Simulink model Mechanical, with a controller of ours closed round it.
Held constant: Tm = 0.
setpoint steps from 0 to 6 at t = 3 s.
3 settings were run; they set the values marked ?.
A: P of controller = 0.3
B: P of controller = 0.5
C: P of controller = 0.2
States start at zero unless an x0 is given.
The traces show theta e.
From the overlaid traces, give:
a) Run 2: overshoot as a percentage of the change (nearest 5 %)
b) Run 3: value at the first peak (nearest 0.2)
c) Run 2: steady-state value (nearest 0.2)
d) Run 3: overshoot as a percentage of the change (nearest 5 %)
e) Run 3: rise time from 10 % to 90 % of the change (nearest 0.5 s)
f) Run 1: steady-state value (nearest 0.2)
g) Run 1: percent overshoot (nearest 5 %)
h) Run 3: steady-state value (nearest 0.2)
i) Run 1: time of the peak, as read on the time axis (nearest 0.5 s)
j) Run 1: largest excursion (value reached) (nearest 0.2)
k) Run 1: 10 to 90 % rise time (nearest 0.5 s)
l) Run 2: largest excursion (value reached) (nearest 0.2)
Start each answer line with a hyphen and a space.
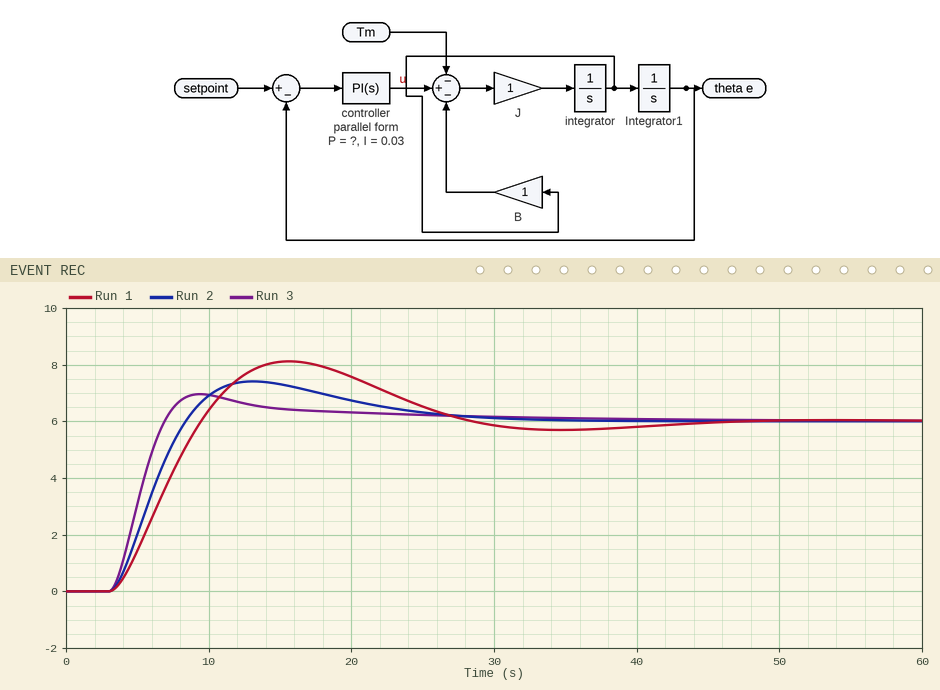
- 25 %
- 7.0
- 6.0
- 15 %
- 2.5 s
- 6.0
- 35 %
- 6.0
- 15.5 s
- 8.2
- 4.5 s
- 7.4
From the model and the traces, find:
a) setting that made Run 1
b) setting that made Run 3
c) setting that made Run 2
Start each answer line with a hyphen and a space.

- C
- B
- A
